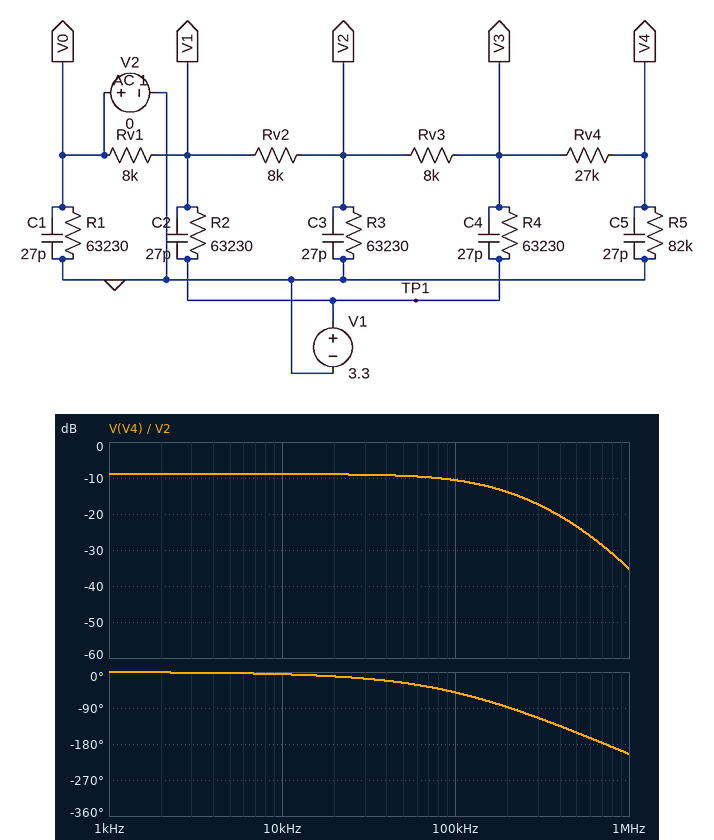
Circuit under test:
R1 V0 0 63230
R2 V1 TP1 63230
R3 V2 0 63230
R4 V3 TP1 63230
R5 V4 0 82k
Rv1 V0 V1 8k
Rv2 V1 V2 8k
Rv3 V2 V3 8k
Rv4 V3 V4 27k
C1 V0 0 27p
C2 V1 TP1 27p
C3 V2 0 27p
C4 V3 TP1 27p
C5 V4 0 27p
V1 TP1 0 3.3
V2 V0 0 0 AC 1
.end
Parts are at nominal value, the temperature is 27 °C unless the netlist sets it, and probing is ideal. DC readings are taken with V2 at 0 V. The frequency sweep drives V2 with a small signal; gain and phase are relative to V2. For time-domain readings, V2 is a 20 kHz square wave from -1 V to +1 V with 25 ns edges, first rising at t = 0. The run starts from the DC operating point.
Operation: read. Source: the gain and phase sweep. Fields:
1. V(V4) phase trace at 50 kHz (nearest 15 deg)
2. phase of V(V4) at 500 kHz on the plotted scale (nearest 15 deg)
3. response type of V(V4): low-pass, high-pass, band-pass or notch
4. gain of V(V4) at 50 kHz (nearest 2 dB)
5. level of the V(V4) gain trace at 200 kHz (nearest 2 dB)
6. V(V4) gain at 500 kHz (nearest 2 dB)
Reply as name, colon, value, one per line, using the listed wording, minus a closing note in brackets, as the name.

V(V4) phase trace at 50 kHz: -30 deg
phase of V(V4) at 500 kHz on the plotted scale: -150 deg
response type of V(V4): low-pass, high-pass, band-pass or notch: low-pass
gain of V(V4) at 50 kHz: -10 dB
level of the V(V4) gain trace at 200 kHz: -14 dB
V(V4) gain at 500 kHz: -24 dB
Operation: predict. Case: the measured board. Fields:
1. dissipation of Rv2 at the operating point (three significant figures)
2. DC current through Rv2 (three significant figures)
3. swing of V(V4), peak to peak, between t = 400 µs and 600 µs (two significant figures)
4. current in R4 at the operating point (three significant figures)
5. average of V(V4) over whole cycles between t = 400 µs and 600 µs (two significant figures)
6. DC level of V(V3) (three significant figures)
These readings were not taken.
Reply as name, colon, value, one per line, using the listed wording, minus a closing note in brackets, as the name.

dissipation of Rv2 at the operating point: 2.97 µW
DC current through Rv2: 19.3 µA
swing of V(V4), peak to peak, between t = 400 µs and 600 µs: 720 mV
current in R4 at the operating point: 38.0 µA
average of V(V4) over whole cycles between t = 400 µs and 600 µs: 680 mV
DC level of V(V3): 899 mV
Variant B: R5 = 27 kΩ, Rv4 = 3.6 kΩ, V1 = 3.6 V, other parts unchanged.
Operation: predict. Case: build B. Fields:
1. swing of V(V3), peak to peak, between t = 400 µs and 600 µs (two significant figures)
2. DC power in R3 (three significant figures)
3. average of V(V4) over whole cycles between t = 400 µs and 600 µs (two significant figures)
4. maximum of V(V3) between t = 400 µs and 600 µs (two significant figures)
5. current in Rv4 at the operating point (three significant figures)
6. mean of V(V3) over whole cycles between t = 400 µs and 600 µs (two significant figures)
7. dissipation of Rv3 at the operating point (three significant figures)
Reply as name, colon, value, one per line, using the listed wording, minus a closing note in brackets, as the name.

swing of V(V3), peak to peak, between t = 400 µs and 600 µs: 720 mV
DC power in R3: 5.31 µW
average of V(V4) over whole cycles between t = 400 µs and 600 µs: 660 mV
maximum of V(V3) between t = 400 µs and 600 µs: 1.1 V
current in Rv4 at the operating point: 24.4 µA
mean of V(V3) over whole cycles between t = 400 µs and 600 µs: 750 mV
dissipation of Rv3 at the operating point: 3.45 µW
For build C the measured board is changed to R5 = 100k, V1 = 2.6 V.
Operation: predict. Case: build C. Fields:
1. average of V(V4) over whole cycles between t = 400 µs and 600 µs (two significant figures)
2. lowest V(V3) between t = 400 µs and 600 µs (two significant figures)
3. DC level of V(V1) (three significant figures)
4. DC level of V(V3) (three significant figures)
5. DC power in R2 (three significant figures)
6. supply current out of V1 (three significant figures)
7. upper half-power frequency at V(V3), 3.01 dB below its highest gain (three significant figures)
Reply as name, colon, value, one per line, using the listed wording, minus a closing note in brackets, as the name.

average of V(V4) over whole cycles between t = 400 µs and 600 µs: 570 mV
lowest V(V3) between t = 400 µs and 600 µs: 240 mV
DC level of V(V1): 403 mV
DC level of V(V3): 721 mV
DC power in R2: 76.3 µW
supply current out of V1: 64.5 µA
upper half-power frequency at V(V3), 3.01 dB below its highest gain: 176 kHz
